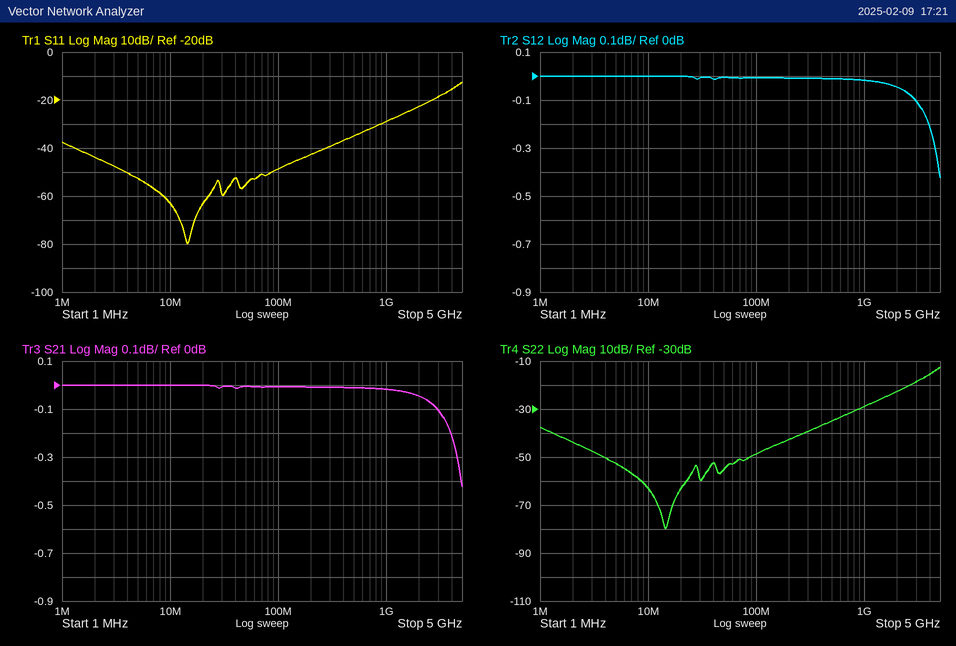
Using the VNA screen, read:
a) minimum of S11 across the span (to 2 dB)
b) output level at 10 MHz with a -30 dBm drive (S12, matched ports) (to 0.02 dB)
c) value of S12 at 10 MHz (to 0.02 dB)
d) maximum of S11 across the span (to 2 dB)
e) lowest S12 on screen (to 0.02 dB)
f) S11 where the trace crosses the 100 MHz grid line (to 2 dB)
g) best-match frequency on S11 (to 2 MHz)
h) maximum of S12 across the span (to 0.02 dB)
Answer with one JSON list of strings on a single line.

["-80 dB", "-30.00 dBm", "0.00 dB", "-12 dB", "-0.42 dB", "-48 dB", "14 MHz", "0.00 dB"]
